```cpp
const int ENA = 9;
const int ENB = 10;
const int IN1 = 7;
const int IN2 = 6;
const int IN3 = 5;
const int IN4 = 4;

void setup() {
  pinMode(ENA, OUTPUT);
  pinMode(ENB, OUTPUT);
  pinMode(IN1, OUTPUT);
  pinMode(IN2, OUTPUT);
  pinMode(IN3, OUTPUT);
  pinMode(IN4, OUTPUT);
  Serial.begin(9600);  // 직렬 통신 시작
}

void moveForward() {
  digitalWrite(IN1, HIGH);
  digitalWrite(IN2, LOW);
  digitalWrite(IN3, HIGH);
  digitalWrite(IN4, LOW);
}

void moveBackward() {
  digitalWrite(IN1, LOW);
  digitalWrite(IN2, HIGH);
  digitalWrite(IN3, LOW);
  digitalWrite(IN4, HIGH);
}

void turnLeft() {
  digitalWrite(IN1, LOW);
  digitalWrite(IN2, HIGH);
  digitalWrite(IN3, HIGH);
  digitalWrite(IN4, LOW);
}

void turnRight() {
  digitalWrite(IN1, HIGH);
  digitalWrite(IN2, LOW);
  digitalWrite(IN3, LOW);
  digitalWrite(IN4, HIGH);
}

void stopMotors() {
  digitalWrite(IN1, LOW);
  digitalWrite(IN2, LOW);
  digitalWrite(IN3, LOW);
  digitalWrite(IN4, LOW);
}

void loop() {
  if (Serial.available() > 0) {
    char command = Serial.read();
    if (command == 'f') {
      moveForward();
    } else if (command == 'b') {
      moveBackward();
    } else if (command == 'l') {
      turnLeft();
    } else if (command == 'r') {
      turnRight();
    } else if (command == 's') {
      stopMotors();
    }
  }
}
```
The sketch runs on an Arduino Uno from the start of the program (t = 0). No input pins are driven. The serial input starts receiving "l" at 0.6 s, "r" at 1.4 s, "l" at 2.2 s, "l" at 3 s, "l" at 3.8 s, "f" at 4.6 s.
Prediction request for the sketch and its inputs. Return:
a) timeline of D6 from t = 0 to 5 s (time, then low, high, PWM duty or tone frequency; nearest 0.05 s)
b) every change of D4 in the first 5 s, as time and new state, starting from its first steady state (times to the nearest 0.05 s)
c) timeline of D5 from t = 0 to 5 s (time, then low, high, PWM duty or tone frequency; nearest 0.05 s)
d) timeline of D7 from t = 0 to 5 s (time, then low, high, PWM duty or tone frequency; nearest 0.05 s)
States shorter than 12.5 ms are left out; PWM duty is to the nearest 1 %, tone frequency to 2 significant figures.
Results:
0 s low; 0.6 s high; 1.4 s low; 2.2 s high; 4.6 s low
0 s low; 1.4 s high; 2.2 s low
0 s low; 0.6 s high; 1.4 s low; 2.2 s high
0 s low; 1.4 s high; 2.2 s low; 4.6 s high
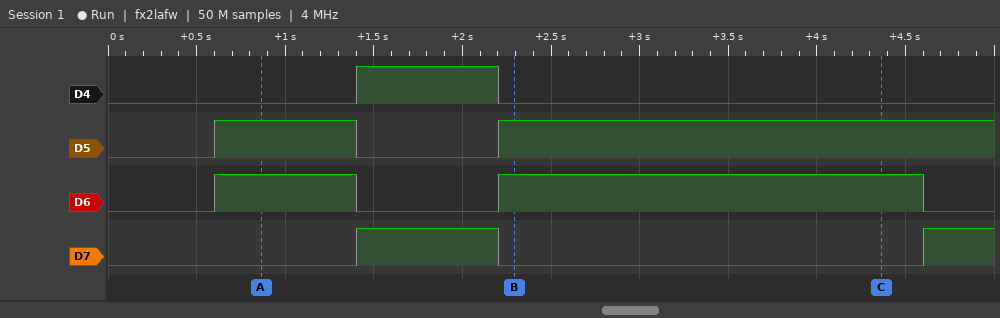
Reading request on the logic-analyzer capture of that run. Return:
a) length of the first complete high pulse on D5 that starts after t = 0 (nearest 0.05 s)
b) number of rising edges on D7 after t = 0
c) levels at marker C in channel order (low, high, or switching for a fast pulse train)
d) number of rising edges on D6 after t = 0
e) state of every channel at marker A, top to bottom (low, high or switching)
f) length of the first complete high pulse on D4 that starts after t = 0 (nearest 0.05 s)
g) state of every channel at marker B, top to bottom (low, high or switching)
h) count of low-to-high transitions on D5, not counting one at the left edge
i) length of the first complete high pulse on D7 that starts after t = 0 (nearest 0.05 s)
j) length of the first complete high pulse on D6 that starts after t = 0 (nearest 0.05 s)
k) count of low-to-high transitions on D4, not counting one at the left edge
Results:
0.80 s
2
D4 low, D5 high, D6 high, D7 low
2
D4 low, D5 high, D6 high, D7 low
0.80 s
D4 low, D5 high, D6 high, D7 low
2
0.80 s
0.80 s
1
